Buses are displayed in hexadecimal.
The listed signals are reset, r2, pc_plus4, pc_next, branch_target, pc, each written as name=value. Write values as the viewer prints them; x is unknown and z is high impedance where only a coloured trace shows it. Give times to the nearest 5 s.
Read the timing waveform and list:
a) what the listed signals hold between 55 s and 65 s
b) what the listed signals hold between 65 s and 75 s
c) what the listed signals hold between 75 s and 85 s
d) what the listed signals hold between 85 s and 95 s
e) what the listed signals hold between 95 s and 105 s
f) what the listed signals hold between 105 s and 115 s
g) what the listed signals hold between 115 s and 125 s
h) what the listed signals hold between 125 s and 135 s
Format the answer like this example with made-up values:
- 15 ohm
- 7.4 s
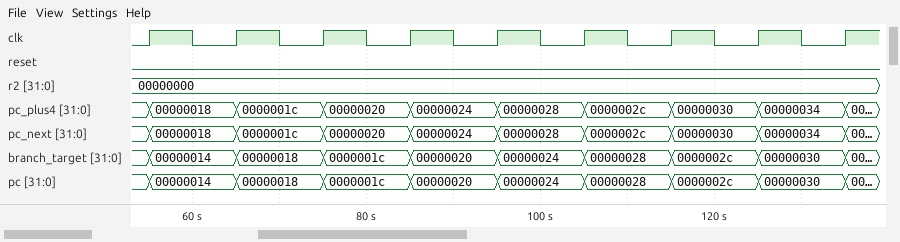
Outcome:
- reset=0, r2=00000000, pc_plus4=00000018, pc_next=00000018, branch_target=00000014, pc=00000014
- reset=0, r2=00000000, pc_plus4=0000001c, pc_next=0000001c, branch_target=00000018, pc=00000018
- reset=0, r2=00000000, pc_plus4=00000020, pc_next=00000020, branch_target=0000001c, pc=0000001c
- reset=0, r2=00000000, pc_plus4=00000024, pc_next=00000024, branch_target=00000020, pc=00000020
- reset=0, r2=00000000, pc_plus4=00000028, pc_next=00000028, branch_target=00000024, pc=00000024
- reset=0, r2=00000000, pc_plus4=0000002c, pc_next=0000002c, branch_target=00000028, pc=00000028
- reset=0, r2=00000000, pc_plus4=00000030, pc_next=00000030, branch_target=0000002c, pc=0000002c
- reset=0, r2=00000000, pc_plus4=00000034, pc_next=00000034, branch_target=00000030, pc=00000030
